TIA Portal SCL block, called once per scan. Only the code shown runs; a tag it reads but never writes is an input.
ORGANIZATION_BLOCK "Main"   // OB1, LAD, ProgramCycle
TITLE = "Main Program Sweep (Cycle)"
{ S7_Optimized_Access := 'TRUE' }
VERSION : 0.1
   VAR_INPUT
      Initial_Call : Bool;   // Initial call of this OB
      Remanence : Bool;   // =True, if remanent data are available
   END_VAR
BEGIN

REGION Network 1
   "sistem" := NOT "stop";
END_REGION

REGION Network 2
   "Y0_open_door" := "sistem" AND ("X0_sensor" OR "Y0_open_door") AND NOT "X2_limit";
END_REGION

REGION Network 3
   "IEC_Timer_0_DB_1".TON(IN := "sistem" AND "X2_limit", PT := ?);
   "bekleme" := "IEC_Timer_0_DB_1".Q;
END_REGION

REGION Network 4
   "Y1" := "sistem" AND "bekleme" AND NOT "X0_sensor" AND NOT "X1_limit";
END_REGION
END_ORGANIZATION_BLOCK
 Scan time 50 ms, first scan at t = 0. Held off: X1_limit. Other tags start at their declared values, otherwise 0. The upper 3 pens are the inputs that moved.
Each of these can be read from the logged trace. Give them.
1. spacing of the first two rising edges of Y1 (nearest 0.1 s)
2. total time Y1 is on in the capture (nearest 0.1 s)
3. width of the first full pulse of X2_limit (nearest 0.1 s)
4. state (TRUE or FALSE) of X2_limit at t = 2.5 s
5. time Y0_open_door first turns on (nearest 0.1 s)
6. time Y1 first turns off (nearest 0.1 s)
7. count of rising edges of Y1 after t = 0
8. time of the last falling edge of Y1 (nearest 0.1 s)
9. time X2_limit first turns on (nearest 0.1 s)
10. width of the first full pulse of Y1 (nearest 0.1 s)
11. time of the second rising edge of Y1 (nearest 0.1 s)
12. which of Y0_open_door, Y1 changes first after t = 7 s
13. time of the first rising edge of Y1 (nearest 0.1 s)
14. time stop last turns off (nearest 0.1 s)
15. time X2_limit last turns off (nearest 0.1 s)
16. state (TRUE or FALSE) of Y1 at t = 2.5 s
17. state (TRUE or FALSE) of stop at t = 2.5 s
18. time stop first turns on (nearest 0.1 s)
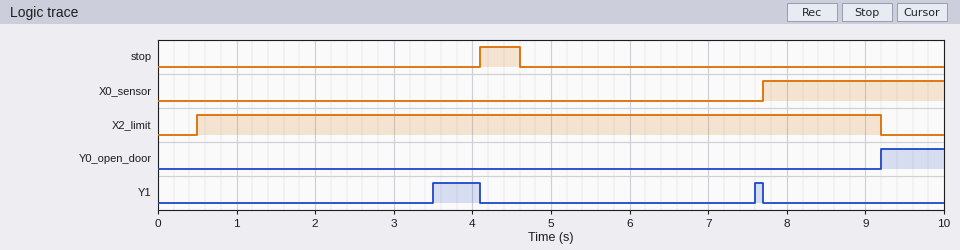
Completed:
4.1 s
0.7 s
8.7 s
TRUE
9.2 s
4.1 s
2
7.7 s
0.5 s
0.6 s
7.6 s
Y1
3.5 s
4.6 s
9.2 s
FALSE
FALSE
4.1 s
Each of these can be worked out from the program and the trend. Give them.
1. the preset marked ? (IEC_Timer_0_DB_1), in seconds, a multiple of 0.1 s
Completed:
3.0 s
